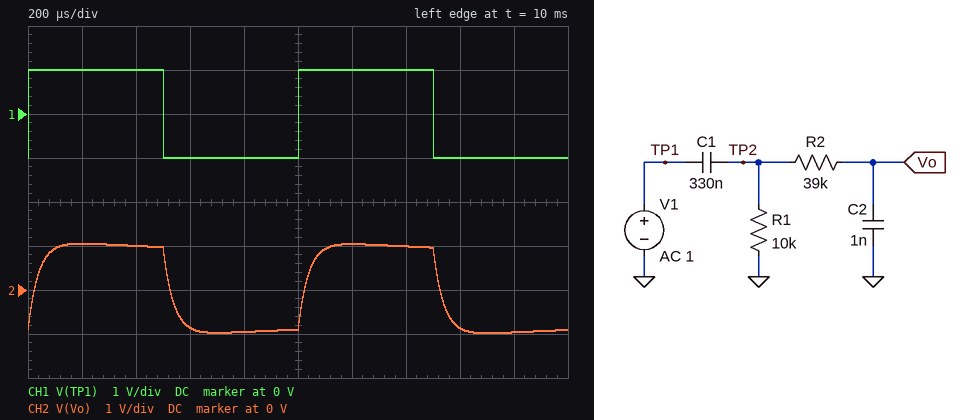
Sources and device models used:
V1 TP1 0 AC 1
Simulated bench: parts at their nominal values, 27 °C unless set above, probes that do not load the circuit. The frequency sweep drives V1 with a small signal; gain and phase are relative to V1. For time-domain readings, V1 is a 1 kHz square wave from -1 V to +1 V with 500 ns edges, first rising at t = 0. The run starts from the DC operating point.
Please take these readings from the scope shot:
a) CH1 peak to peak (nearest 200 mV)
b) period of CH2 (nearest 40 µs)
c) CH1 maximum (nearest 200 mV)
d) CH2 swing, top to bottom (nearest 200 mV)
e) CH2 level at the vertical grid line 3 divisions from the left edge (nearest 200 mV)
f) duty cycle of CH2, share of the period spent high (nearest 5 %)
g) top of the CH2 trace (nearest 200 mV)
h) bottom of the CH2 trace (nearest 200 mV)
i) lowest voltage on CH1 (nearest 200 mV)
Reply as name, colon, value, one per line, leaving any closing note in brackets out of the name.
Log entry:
CH1 peak to peak: 2.0 V
period of CH2: 1.00 ms
CH1 maximum: 1.0 V
CH2 swing, top to bottom: 2.0 V
CH2 level at the vertical grid line 3 divisions from the left edge: -800 mV
duty cycle of CH2, share of the period spent high: 50 %
top of the CH2 trace: 1.0 V
bottom of the CH2 trace: -1.0 V
lowest voltage on CH1: -1.0 V
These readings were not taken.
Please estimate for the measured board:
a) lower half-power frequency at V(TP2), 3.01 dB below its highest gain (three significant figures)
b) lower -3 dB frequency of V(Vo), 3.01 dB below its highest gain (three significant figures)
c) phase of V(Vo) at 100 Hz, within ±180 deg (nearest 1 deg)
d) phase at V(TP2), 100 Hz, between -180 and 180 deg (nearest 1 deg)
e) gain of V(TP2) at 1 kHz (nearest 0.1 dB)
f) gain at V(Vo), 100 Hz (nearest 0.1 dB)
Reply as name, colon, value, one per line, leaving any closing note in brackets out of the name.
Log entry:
lower half-power frequency at V(TP2), 3.01 dB below its highest gain: 48.4 Hz
lower -3 dB frequency of V(Vo), 3.01 dB below its highest gain: 47.0 Hz
phase of V(Vo) at 100 Hz, within ±180 deg: 24 deg
phase at V(TP2), 100 Hz, between -180 and 180 deg: 26 deg
gain of V(TP2) at 1 kHz: 0 dB
gain at V(Vo), 100 Hz: -0.9 dB
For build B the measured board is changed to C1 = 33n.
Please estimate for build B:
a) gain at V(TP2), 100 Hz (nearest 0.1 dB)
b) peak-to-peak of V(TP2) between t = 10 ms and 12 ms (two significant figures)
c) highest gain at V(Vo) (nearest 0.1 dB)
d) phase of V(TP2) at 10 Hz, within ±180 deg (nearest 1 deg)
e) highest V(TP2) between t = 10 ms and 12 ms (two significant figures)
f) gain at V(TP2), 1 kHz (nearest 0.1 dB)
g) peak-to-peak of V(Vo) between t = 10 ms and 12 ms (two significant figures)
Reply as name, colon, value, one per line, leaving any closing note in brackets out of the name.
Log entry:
gain at V(TP2), 100 Hz: -13.9 dB
peak-to-peak of V(TP2) between t = 10 ms and 12 ms: 3.3 V
highest gain at V(Vo): -1.2 dB
phase of V(TP2) at 10 Hz, within ±180 deg: 89 deg
highest V(TP2) between t = 10 ms and 12 ms: 1.6 V
gain at V(TP2), 1 kHz: -1.1 dB
peak-to-peak of V(Vo) between t = 10 ms and 12 ms: 2.3 V
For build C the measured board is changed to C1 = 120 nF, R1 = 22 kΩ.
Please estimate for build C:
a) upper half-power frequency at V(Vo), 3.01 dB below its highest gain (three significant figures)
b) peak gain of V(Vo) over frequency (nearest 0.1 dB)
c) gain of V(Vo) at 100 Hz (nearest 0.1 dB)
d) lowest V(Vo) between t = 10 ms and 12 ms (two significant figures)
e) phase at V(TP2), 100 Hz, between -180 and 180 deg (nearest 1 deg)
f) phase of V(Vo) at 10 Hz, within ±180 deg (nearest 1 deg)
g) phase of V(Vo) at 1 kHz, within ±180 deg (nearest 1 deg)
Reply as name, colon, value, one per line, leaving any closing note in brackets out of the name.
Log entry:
upper half-power frequency at V(Vo), 3.01 dB below its highest gain: 4.23 kHz
peak gain of V(Vo) over frequency: -0.2 dB
gain of V(Vo) at 100 Hz: -1.4 dB
lowest V(Vo) between t = 10 ms and 12 ms: -1.0 V
phase at V(TP2), 100 Hz, between -180 and 180 deg: 31 deg
phase of V(Vo) at 10 Hz, within ±180 deg: 80 deg
phase of V(Vo) at 1 kHz, within ±180 deg: -10 deg
